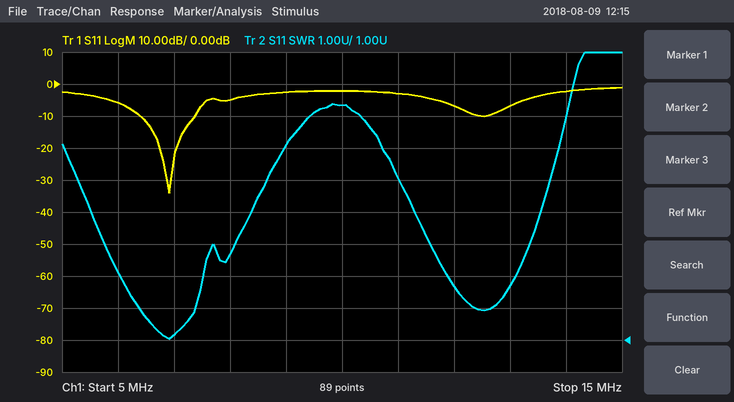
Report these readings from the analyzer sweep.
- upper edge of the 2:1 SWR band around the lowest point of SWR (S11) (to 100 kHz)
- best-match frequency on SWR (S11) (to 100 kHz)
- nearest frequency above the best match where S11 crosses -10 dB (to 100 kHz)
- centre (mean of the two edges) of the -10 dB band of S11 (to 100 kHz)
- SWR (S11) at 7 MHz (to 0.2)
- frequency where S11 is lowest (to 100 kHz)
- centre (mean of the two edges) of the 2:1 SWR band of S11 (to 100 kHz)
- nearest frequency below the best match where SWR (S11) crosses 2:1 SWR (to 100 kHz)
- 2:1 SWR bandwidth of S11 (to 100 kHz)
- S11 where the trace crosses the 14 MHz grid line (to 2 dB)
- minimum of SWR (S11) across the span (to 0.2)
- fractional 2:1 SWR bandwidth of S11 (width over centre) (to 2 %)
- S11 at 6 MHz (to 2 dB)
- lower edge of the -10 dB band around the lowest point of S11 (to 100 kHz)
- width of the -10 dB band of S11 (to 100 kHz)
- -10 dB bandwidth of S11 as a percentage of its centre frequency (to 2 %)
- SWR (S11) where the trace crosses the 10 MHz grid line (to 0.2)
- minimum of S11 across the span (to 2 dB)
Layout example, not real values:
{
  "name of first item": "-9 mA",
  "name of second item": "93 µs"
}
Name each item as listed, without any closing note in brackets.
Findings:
{
  "upper edge of the 2:1 SWR band around the lowest point of SWR (S11)": "7.4 MHz",
  "best-match frequency on SWR (S11)": "6.9 MHz",
  "nearest frequency above the best match where S11 crosses -10 dB": "7.4 MHz",
  "centre (mean of the two edges) of the -10 dB band of S11": "6.9 MHz",
  "SWR (S11) at 7 MHz": "1.2",
  "frequency where S11 is lowest": "6.9 MHz",
  "centre (mean of the two edges) of the 2:1 SWR band of S11": "6.9 MHz",
  "nearest frequency below the best match where SWR (S11) crosses 2:1 SWR": "6.4 MHz",
  "2:1 SWR bandwidth of S11": "1.0 MHz",
  "S11 where the trace crosses the 14 MHz grid line": "-2 dB",
  "minimum of SWR (S11) across the span": "1.0",
  "fractional 2:1 SWR bandwidth of S11 (width over centre)": "14 %",
  "S11 at 6 MHz": "-6 dB",
  "lower edge of the -10 dB band around the lowest point of S11": "6.4 MHz",
  "width of the -10 dB band of S11": "1.0 MHz",
  "-10 dB bandwidth of S11 as a percentage of its centre frequency": "14 %",
  "SWR (S11) where the trace crosses the 10 MHz grid line": "8.4",
  "minimum of S11 across the span": "-34 dB"
}
